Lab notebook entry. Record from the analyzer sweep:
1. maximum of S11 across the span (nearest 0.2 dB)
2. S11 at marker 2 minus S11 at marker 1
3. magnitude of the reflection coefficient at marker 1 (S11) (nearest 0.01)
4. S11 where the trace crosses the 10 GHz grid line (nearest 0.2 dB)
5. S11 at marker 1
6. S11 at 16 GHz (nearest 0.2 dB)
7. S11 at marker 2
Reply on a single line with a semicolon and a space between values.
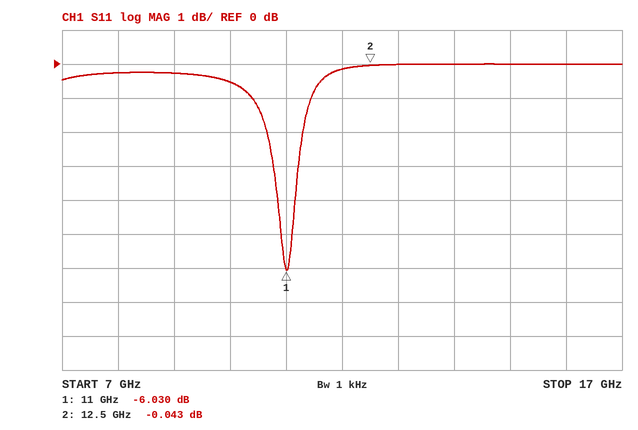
0.0 dB; 5.987 dB; 0.50; -0.6 dB; -6.030 dB; 0.0 dB; -0.043 dB
